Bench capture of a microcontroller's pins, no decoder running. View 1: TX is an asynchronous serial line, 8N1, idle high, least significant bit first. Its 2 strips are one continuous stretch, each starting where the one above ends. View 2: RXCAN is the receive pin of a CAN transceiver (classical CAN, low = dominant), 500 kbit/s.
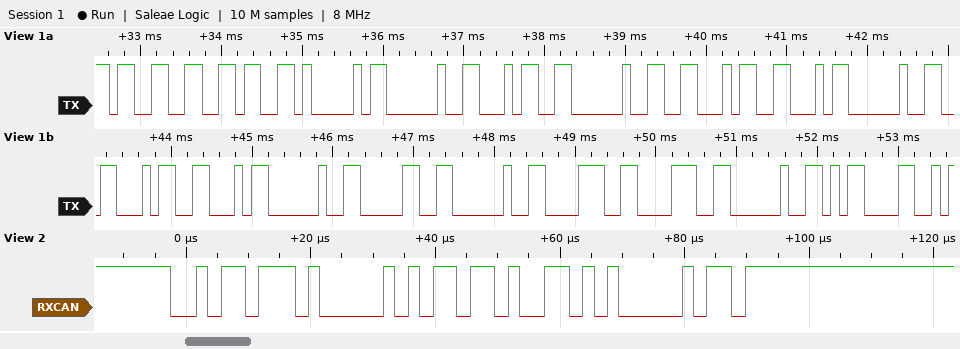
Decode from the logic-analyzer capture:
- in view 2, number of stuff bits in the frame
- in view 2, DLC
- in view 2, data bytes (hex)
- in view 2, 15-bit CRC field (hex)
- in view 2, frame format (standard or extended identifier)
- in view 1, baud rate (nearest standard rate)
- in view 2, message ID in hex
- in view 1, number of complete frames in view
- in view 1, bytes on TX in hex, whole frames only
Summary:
2
1
6D
0x1A81
standard
9600 baud
0x2DD
18
33 36 41 20 34 20 46 46 20 46 46 20 30 20 38 38 20 0D
